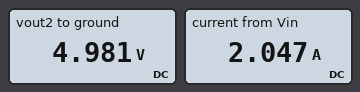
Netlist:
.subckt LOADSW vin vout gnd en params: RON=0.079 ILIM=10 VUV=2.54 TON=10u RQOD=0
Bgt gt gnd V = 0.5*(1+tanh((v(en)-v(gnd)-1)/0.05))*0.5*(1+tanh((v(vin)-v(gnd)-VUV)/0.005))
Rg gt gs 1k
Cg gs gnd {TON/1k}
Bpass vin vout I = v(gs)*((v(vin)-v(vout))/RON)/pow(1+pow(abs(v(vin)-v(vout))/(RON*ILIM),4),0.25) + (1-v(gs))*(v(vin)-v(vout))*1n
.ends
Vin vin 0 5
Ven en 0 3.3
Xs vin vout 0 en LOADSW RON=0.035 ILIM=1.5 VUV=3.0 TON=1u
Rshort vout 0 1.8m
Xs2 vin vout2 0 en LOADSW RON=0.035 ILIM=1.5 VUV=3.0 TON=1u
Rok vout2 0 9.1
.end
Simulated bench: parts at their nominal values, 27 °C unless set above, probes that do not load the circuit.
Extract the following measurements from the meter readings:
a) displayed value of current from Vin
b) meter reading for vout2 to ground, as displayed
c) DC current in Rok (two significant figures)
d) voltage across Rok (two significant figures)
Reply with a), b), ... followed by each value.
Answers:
a) 2.047 A
b) 4.981 V
c) 550 mA
d) 5.0 V
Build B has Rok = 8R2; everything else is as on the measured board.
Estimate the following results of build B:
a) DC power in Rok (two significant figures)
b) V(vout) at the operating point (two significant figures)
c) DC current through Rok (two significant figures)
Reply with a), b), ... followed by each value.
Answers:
a) 3.0 W
b) 2.7 mV
c) 610 mA
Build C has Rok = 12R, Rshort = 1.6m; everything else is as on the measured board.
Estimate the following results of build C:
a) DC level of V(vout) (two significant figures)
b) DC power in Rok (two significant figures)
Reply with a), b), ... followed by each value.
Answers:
a) 2.4 mV
b) 2.1 W
